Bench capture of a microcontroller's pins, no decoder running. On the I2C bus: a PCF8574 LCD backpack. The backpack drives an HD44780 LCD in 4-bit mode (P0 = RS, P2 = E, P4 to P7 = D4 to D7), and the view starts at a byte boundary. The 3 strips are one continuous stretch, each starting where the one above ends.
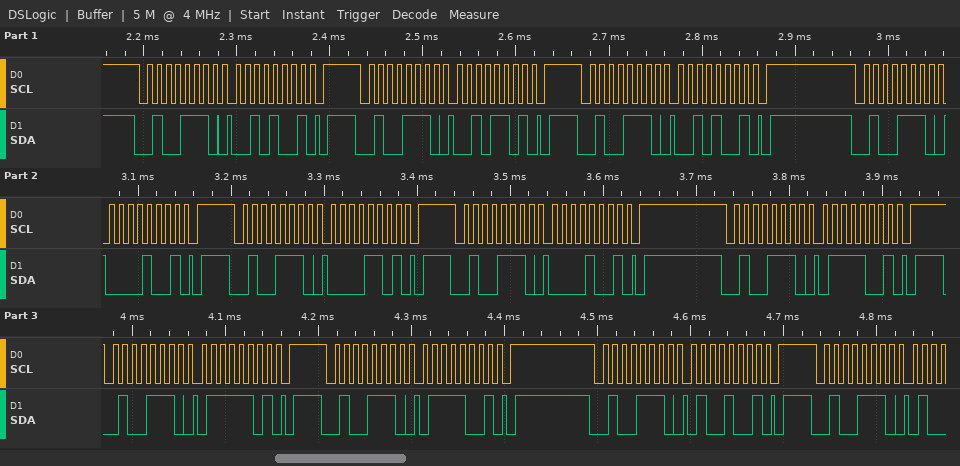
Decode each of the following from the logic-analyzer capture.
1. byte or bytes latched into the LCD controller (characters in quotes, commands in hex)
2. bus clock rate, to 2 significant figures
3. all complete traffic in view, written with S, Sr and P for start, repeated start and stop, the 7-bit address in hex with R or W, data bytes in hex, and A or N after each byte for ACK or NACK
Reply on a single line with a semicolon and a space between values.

' '; 100 kHz; S 27W A 29 A P S 27W A 2D A P S 27W A 29 A P S 27W A 09 A P S 27W A 0D A P S 27W A 09 A P S 27W A 79 A P S 27W A 7D A P S 27W A 79 A P S 27W A 49 A P S 27W A
